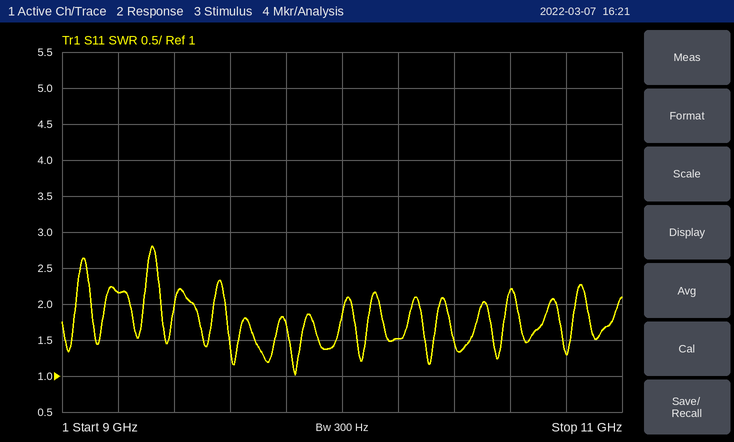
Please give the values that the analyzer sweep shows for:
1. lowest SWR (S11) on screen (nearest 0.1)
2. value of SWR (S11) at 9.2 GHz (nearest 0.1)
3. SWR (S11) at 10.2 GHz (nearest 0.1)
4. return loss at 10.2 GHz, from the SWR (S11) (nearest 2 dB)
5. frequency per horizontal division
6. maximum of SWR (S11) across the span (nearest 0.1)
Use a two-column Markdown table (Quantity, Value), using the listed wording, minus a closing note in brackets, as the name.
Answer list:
| Quantity | Value |
|---|---|
| lowest SWR (S11) on screen | 1.0 |
| value of SWR (S11) at 9.2 GHz | 2.2 |
| SWR (S11) at 10.2 GHz | 1.5 |
| return loss at 10.2 GHz, from the SWR (S11) | 14 dB |
| frequency per horizontal division | 200 MHz |
| maximum of SWR (S11) across the span | 2.8 |
